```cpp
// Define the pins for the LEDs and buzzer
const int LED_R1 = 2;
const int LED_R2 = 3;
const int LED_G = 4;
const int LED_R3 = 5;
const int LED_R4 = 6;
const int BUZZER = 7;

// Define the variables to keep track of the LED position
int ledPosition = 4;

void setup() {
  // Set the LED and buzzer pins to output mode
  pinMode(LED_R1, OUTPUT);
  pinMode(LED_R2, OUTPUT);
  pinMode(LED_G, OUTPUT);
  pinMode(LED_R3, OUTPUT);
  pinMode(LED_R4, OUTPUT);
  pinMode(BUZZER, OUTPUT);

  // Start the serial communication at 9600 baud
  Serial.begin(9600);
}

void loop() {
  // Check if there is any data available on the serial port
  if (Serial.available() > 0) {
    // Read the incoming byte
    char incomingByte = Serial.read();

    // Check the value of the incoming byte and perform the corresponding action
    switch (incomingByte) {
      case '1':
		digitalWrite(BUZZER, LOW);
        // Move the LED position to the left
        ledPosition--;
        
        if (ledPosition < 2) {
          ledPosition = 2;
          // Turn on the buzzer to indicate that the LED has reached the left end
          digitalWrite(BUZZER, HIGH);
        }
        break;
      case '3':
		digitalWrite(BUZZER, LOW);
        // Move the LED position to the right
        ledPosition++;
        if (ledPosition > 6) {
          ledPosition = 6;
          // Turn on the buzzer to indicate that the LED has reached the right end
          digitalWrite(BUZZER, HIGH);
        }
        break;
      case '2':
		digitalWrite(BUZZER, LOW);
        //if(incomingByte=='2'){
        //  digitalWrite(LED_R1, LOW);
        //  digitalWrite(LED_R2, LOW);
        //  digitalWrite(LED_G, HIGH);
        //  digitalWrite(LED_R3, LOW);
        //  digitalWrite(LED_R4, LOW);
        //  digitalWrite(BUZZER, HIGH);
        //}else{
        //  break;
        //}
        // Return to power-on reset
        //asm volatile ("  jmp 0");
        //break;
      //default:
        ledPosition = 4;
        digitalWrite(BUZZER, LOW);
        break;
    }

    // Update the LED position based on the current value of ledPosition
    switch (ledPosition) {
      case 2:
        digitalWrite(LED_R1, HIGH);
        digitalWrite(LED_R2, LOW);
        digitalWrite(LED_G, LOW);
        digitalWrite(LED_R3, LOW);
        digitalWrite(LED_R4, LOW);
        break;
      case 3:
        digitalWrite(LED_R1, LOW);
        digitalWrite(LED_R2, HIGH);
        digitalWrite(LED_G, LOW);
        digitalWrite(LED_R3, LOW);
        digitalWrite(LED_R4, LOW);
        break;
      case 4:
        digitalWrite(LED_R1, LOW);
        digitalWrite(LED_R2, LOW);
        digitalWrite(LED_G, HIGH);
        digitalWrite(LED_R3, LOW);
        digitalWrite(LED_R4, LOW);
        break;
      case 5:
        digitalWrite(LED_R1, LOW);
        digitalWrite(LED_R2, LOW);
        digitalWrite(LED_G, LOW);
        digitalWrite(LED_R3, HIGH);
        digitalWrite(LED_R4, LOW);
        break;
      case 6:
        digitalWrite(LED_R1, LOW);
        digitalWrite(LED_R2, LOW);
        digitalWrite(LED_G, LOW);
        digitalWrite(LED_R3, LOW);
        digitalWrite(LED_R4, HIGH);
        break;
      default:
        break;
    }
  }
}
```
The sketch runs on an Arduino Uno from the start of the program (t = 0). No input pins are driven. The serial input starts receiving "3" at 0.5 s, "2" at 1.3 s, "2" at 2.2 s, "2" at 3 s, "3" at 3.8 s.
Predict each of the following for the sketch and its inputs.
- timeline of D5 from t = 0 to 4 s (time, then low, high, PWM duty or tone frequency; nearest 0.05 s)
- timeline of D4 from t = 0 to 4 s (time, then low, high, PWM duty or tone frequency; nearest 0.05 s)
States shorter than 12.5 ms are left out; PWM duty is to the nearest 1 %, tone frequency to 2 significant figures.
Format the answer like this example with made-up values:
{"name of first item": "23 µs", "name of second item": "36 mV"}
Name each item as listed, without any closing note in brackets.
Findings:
{"timeline of D5 from t = 0 to 4 s": "0 s low; 0.5 s high; 1.3 s low; 3.8 s high", "timeline of D4 from t = 0 to 4 s": "0 s low; 1.3 s high; 3.8 s low"}
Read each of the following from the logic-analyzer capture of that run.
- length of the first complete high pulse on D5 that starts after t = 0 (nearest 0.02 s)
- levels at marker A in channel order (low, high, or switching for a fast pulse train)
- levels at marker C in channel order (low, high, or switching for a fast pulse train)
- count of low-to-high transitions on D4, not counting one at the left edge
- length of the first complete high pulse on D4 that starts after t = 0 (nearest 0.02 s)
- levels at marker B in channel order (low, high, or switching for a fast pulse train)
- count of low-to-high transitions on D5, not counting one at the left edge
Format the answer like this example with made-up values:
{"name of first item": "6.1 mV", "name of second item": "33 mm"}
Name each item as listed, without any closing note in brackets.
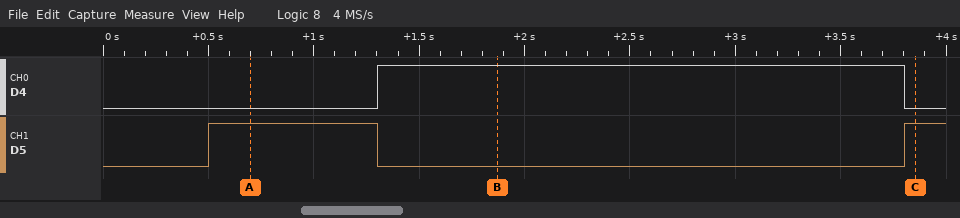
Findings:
{"length of the first complete high pulse on D5 that starts after t = 0": "0.80 s", "levels at marker A in channel order": "D4 low, D5 high", "levels at marker C in channel order": "D4 low, D5 high", "count of low-to-high transitions on D4, not counting one at the left edge": "1", "length of the first complete high pulse on D4 that starts after t = 0": "2.50 s", "levels at marker B in channel order": "D4 high, D5 low", "count of low-to-high transitions on D5, not counting one at the left edge": "2"}
